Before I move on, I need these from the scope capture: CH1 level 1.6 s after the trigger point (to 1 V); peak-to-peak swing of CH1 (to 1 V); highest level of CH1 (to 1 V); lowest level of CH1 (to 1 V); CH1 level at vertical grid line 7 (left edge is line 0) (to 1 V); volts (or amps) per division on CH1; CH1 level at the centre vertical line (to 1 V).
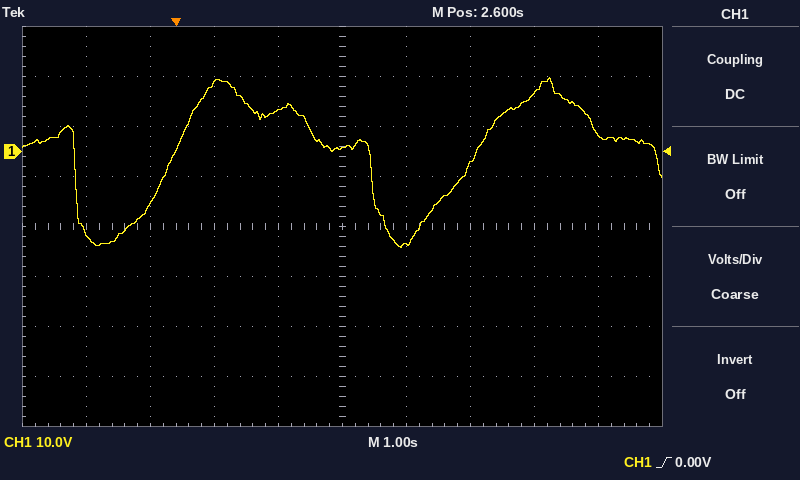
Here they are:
8 V
34 V
15 V
-19 V
-3 V
10 V
1 V
